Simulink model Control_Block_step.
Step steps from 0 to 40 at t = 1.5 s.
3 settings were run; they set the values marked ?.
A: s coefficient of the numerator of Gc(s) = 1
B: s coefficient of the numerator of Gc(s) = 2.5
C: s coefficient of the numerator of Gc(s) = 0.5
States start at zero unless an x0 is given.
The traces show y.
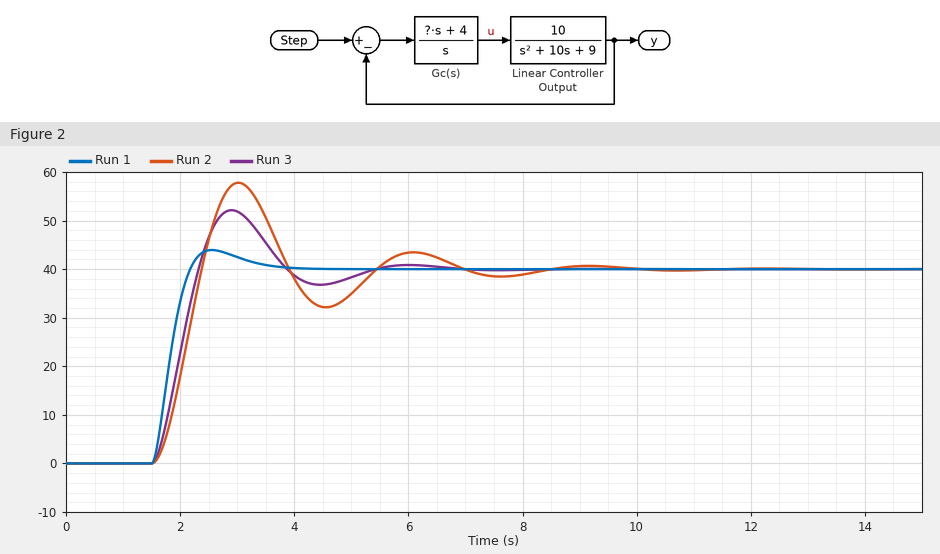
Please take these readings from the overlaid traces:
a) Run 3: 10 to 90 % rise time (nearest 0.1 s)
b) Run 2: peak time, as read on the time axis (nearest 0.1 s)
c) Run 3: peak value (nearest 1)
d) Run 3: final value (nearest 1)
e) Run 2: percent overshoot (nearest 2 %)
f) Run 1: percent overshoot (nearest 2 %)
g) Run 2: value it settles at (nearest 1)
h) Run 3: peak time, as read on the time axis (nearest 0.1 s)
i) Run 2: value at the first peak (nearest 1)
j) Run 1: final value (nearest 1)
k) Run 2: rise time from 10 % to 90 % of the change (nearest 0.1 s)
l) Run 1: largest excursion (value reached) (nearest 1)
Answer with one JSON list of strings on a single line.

["0.6 s", "3.0 s", "52", "40", "44 %", "10 %", "40", "2.9 s", "58", "40", "0.6 s", "44"]
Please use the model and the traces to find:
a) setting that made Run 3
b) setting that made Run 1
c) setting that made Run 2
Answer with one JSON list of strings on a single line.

["A", "B", "C"]
